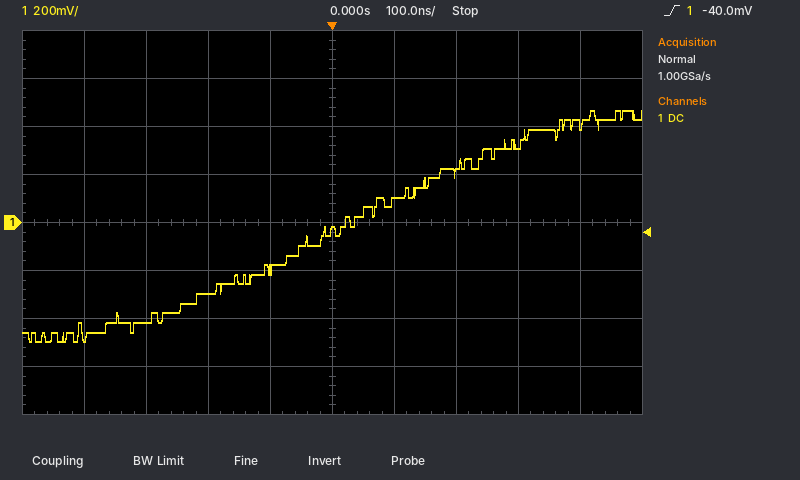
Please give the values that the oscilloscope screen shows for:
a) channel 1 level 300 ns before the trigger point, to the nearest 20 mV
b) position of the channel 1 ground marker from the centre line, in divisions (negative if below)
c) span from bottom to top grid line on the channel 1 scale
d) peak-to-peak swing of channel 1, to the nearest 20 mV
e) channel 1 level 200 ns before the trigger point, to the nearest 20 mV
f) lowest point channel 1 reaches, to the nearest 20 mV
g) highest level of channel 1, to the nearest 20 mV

-420 mV
0.0 div
1.6 V
960 mV
-300 mV
-500 mV
460 mV
